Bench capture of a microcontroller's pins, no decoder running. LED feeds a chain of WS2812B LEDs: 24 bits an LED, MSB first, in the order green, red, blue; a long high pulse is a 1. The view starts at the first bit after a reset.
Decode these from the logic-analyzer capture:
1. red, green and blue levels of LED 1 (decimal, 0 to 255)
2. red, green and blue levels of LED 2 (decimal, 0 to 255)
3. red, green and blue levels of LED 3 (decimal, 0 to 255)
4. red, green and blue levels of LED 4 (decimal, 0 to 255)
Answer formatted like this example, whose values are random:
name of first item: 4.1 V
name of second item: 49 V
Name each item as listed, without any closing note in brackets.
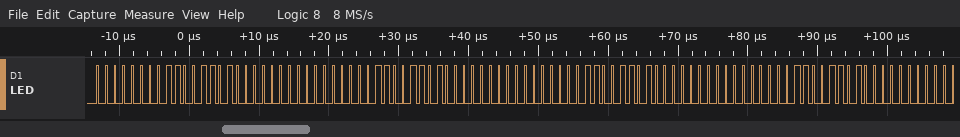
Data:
red, green and blue levels of LED 1: 205, 0, 0
red, green and blue levels of LED 2: 205, 0, 0
red, green and blue levels of LED 3: 205, 0, 0
red, green and blue levels of LED 4: 205, 0, 0
